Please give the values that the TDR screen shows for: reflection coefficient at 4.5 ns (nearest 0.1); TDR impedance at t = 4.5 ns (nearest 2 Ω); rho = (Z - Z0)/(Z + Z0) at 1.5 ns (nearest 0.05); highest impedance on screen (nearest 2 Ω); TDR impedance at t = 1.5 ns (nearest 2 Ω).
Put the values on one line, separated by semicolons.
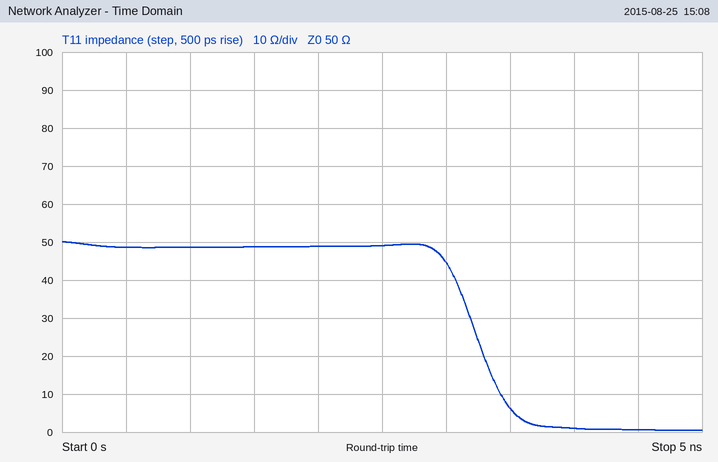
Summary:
-1.0; 0 Ω; 0.00; 50 Ω; 48 Ω
